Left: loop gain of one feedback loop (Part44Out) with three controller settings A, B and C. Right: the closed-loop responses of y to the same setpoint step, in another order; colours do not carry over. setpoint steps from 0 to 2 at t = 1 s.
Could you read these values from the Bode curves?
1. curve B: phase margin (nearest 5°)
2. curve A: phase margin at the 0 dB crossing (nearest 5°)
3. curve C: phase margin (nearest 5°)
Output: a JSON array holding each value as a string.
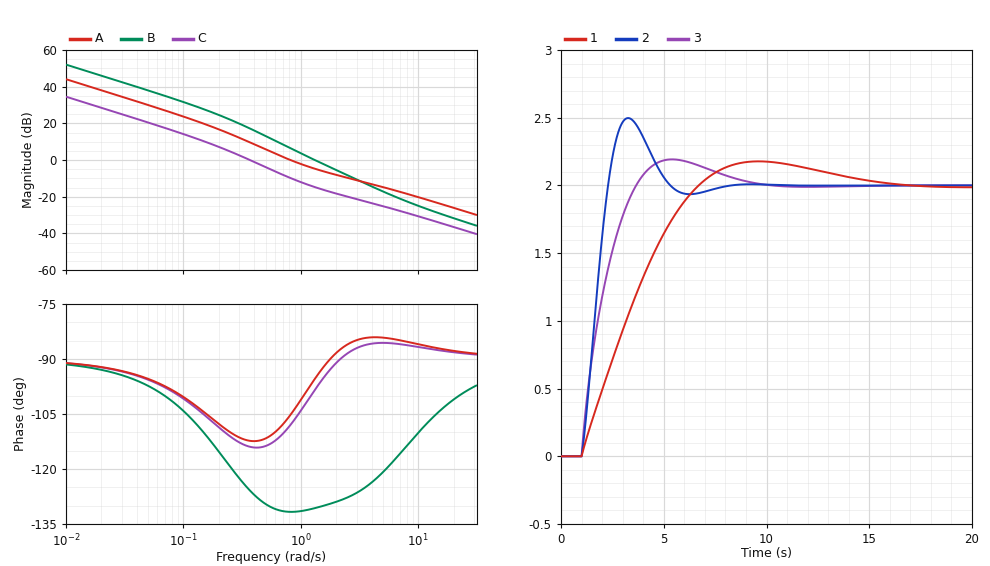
["50°", "75°", "65°"]
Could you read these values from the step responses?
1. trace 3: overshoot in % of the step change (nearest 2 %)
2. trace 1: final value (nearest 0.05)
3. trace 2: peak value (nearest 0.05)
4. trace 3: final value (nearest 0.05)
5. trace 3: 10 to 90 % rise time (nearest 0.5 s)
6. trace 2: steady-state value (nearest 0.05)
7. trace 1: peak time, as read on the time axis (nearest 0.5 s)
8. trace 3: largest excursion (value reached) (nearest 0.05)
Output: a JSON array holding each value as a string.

["10 %", "2.00", "2.50", "2.00", "2.0 s", "2.00", "9.5 s", "2.20"]
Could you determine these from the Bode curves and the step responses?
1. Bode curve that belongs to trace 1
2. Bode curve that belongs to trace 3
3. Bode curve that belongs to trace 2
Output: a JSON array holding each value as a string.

["C", "A", "B"]
